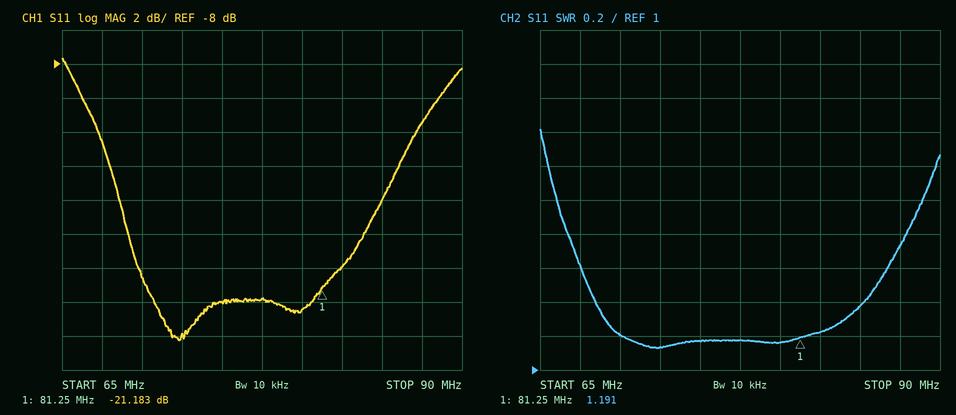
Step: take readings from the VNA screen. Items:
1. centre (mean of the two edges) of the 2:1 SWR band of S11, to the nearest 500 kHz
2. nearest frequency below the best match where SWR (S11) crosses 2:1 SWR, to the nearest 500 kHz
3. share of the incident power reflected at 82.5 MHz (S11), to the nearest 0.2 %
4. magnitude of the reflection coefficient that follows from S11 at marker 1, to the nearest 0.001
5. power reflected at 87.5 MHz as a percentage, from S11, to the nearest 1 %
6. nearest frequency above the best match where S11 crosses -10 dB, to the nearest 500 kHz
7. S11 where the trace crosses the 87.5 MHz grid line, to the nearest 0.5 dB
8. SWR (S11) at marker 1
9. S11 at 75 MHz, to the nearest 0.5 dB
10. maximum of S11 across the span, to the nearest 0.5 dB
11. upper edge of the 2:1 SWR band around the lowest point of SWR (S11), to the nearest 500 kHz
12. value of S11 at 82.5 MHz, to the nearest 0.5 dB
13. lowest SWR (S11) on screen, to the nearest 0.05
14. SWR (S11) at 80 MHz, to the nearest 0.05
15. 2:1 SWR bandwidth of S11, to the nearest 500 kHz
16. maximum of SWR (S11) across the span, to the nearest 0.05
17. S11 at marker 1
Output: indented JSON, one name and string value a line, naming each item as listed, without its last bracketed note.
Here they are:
{
  "centre (mean of the two edges) of the 2:1 SWR band of S11, to the nearest 500 kHz": "77.5 MHz",
  "nearest frequency below the best match where SWR (S11) crosses 2:1 SWR, to the nearest 500 kHz": "66.0 MHz",
  "share of the incident power reflected at 82.5 MHz (S11), to the nearest 0.2 %": "1.0 %",
  "magnitude of the reflection coefficient that follows from S11 at marker 1, to the nearest 0.001": "0.087",
  "power reflected at 87.5 MHz as a percentage, from S11, to the nearest 1 %": "7 %",
  "nearest frequency above the best match where S11 crosses -10 dB, to the nearest 500 kHz": "88.5 MHz",
  "S11 where the trace crosses the 87.5 MHz grid line, to the nearest 0.5 dB": "-11.5 dB",
  "SWR (S11) at marker 1": "1.191",
  "S11 at 75 MHz, to the nearest 0.5 dB": "-22.0 dB",
  "maximum of S11 across the span, to the nearest 0.5 dB": "-7.5 dB",
  "upper edge of the 2:1 SWR band around the lowest point of SWR (S11), to the nearest 500 kHz": "89.0 MHz",
  "value of S11 at 82.5 MHz, to the nearest 0.5 dB": "-20.0 dB",
  "lowest SWR (S11) on screen, to the nearest 0.05": "1.15",
  "SWR (S11) at 80 MHz, to the nearest 0.05": "1.15",
  "2:1 SWR bandwidth of S11, to the nearest 500 kHz": "23.0 MHz",
  "maximum of SWR (S11) across the span, to the nearest 0.05": "2.40",
  "S11 at marker 1": "-21.183 dB"
}
